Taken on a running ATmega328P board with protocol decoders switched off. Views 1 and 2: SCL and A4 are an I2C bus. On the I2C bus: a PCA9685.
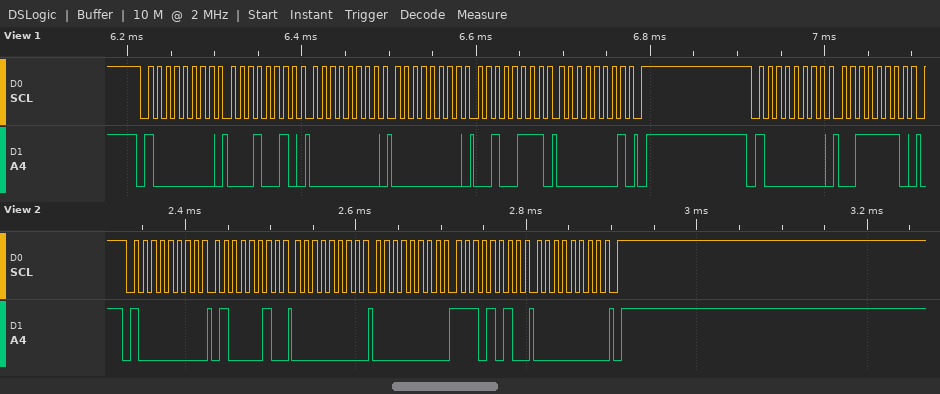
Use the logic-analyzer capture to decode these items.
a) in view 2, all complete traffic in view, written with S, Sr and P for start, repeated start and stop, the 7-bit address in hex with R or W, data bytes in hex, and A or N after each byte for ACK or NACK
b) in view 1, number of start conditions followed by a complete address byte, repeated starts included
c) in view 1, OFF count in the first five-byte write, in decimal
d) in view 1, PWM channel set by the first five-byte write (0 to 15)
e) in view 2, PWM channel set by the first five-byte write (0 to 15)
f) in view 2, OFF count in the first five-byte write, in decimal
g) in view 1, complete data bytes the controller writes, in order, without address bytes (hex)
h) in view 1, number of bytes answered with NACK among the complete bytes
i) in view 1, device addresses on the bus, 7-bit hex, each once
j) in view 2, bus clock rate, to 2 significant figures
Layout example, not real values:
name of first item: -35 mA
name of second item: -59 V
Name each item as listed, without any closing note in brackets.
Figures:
in view 2, all complete traffic in view, written with S, Sr and P for start, repeated start and stop, the 7-bit address in hex with R or W, data bytes in hex, and A or N after each byte for ACK or NACK: S 40W A 42 A 00 A 00 A EA A 00 A P
in view 1, number of start conditions followed by a complete address byte, repeated starts included: 2
in view 1, OFF count in the first five-byte write, in decimal: 295
in view 1, PWM channel set by the first five-byte write: 3
in view 2, PWM channel set by the first five-byte write: 15
in view 2, OFF count in the first five-byte write, in decimal: 234
in view 1, complete data bytes the controller writes, in order, without address bytes: 12 00 00 27 01 3E
in view 1, number of bytes answered with NACK among the complete bytes: 0
in view 1, device addresses on the bus, 7-bit hex, each once: 0x40
in view 2, bus clock rate, to 2 significant figures: 100 kHz
